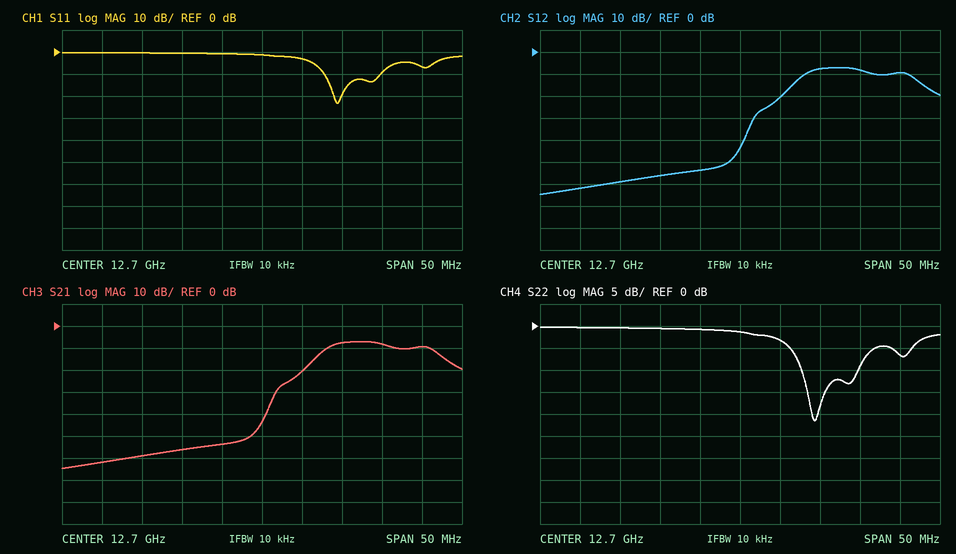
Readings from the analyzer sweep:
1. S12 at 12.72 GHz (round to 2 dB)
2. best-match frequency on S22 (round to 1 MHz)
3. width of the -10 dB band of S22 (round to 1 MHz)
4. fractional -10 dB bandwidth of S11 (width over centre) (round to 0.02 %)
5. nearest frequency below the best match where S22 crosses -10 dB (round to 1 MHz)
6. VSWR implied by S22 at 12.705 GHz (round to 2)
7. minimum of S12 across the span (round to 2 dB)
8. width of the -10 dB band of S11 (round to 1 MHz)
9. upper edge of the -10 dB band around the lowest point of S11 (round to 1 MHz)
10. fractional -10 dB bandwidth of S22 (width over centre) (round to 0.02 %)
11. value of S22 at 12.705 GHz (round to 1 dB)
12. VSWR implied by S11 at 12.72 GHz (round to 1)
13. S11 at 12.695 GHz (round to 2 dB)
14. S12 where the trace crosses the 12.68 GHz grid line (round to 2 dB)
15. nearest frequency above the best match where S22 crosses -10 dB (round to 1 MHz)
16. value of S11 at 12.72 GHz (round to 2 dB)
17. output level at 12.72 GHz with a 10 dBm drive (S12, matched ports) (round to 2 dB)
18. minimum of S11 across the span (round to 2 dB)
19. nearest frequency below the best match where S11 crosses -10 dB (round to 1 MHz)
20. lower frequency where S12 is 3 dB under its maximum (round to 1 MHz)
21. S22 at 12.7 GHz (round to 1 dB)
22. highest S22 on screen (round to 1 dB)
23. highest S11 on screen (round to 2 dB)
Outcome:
-10 dB
12.709 GHz
7 MHz
0.06 %
12.708 GHz
6
-64 dB
7 MHz
12.715 GHz
0.06 %
-3 dB
3
0 dB
-62 dB
12.715 GHz
-6 dB
0 dBm
-24 dB
12.708 GHz
12.708 GHz
-1 dB
0 dB
0 dB
